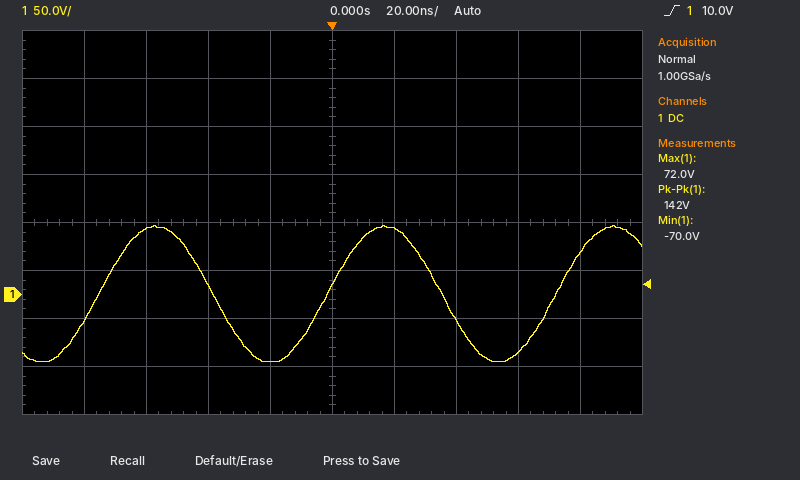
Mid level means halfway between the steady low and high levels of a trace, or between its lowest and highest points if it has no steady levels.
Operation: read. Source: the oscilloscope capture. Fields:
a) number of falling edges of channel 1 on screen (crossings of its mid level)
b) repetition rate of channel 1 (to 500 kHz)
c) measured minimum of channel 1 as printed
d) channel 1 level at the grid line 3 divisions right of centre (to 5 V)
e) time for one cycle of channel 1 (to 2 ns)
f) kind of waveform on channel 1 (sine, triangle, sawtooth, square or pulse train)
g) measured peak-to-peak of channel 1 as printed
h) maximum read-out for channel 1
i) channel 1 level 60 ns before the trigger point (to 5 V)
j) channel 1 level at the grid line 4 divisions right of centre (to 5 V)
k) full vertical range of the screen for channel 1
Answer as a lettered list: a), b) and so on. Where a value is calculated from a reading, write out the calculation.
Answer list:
a) 2
b) 1 / 74 ns ≈ 13.5 MHz
c) -70.0 V
d) -60 V
e) 74 ns
f) sine
g) 142 V
h) 72.0 V
i) 70 V
j) 45 V
k) 400 V
